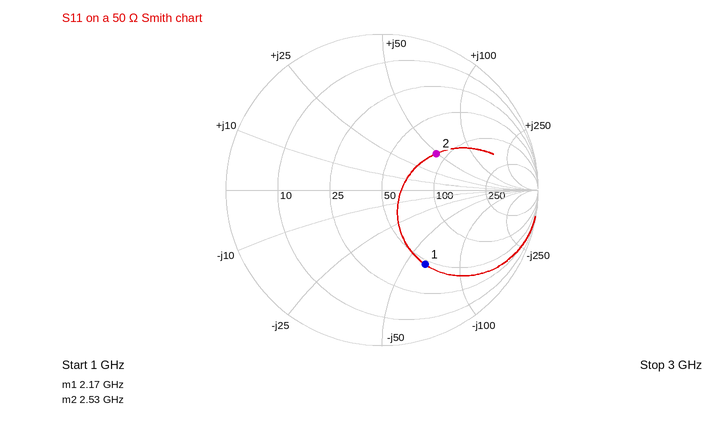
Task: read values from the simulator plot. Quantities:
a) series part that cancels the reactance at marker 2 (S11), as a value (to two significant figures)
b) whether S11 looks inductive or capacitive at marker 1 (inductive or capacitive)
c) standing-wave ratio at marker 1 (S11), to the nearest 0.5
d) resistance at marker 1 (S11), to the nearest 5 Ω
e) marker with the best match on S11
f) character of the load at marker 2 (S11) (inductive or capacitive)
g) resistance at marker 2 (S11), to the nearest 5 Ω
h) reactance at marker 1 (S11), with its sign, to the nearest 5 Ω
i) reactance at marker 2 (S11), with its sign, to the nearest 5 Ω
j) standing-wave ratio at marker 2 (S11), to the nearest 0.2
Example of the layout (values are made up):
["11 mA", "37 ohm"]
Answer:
["1.3 pF", "capacitive", "3.5", "45 Ω", "marker 2", "inductive", "85 Ω", "-65 Ω", "+50 Ω", "2.4"]
